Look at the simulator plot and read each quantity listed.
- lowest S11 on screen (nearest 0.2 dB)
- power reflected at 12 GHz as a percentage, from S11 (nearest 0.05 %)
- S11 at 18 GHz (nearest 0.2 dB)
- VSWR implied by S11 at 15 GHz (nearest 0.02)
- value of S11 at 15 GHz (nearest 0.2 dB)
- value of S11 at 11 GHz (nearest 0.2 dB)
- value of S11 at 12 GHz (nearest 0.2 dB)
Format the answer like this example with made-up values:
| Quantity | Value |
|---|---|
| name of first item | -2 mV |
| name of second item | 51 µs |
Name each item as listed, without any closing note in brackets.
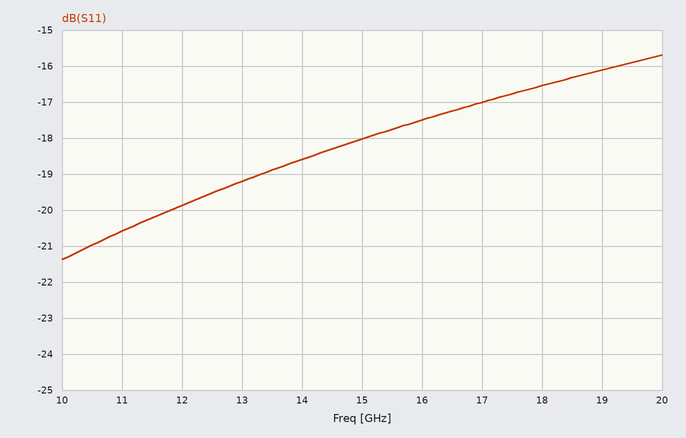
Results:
| Quantity | Value |
|---|---|
| lowest S11 on screen | -21.4 dB |
| power reflected at 12 GHz as a percentage, from S11 | 1.05 % |
| S11 at 18 GHz | -16.6 dB |
| VSWR implied by S11 at 15 GHz | 1.28 |
| value of S11 at 15 GHz | -18.0 dB |
| value of S11 at 11 GHz | -20.6 dB |
| value of S11 at 12 GHz | -19.8 dB |
